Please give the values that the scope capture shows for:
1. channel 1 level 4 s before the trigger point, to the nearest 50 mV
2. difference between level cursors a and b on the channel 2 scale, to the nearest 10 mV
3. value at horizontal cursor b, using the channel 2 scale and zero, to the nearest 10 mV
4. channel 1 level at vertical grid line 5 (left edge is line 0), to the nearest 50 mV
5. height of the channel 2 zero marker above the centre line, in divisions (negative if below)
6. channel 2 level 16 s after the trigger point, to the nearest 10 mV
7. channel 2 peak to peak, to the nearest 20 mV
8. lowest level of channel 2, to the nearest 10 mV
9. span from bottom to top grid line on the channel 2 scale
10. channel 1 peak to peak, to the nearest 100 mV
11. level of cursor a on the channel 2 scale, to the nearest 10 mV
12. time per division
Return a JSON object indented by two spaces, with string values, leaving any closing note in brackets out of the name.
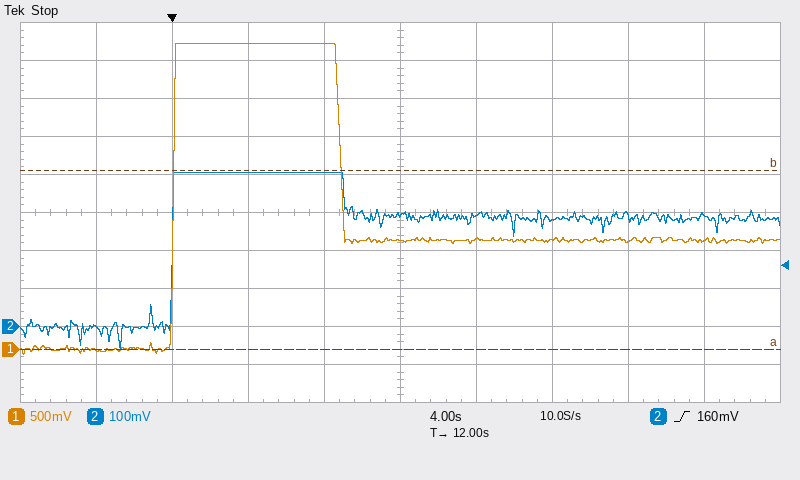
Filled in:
{
  "channel 1 level 4 s before the trigger point, to the nearest 50 mV": "0 mV",
  "difference between level cursors a and b on the channel 2 scale, to the nearest 10 mV": "470 mV",
  "value at horizontal cursor b, using the channel 2 scale and zero, to the nearest 10 mV": "410 mV",
  "channel 1 level at vertical grid line 5 (left edge is line 0), to the nearest 50 mV": "1.45 V",
  "height of the channel 2 zero marker above the centre line, in divisions": "-3.0 div",
  "channel 2 level 16 s after the trigger point, to the nearest 10 mV": "290 mV",
  "channel 2 peak to peak, to the nearest 20 mV": "460 mV",
  "lowest level of channel 2, to the nearest 10 mV": "-60 mV",
  "span from bottom to top grid line on the channel 2 scale": "1 V",
  "channel 1 peak to peak, to the nearest 100 mV": "4.10 V",
  "level of cursor a on the channel 2 scale, to the nearest 10 mV": "-60 mV",
  "time per division": "4 s"
}
